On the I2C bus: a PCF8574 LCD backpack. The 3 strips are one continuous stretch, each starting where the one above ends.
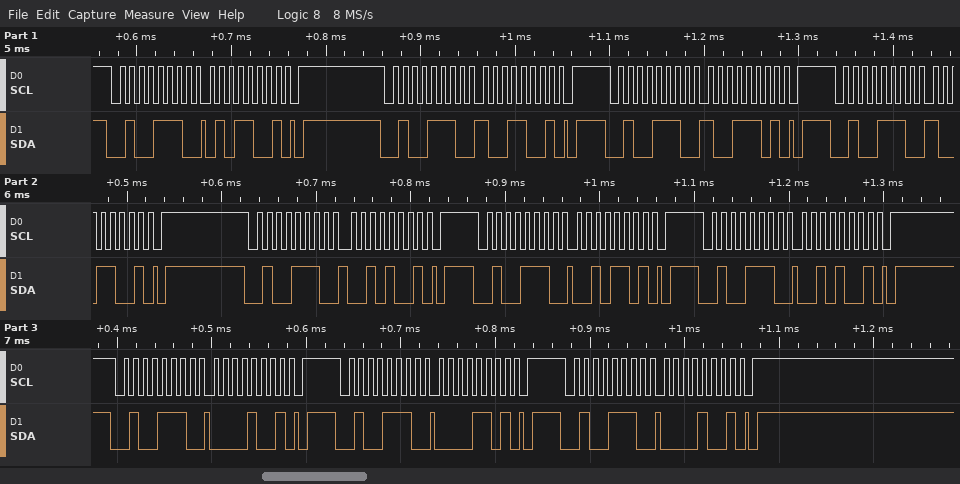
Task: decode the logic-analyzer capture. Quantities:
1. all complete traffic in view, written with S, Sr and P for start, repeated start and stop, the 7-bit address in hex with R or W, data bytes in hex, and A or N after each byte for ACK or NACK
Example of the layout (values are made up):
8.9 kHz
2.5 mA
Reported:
S 27W A 59 A P S 27W A 99 A P S 27W A 9D A P S 27W A 99 A P S 27W A 29 A P S 27W A 2D A P S 27W A 29 A P S 27W A 09 A P S 27W A 0D A P S 27W A 09 A P
